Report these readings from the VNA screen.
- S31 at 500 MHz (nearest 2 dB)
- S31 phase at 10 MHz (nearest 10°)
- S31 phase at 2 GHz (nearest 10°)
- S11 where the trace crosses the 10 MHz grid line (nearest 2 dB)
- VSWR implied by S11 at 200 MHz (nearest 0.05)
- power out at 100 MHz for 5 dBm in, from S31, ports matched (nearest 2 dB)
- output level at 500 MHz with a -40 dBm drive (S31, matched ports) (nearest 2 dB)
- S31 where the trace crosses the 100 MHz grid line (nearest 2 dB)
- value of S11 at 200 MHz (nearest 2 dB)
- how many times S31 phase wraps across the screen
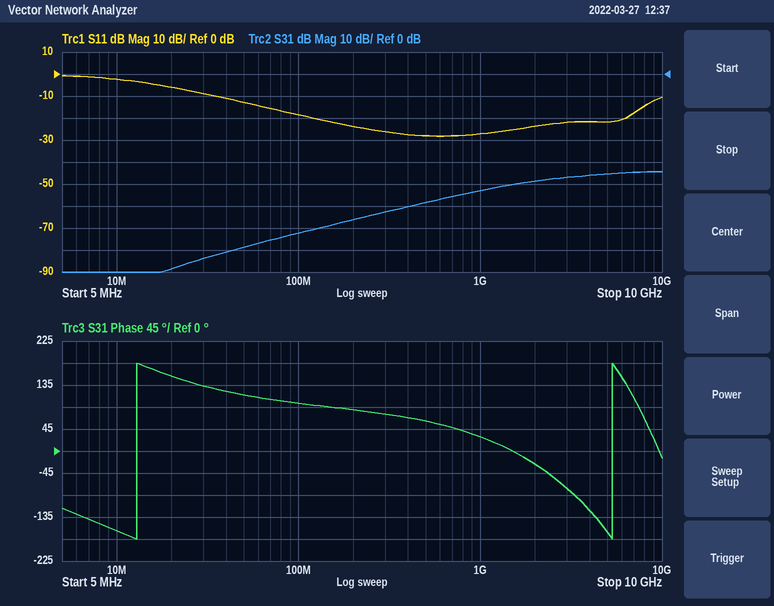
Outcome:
-58 dB
-160°
-30°
-2 dB
1.15
-68 dBm
-98 dBm
-72 dB
-24 dB
2
